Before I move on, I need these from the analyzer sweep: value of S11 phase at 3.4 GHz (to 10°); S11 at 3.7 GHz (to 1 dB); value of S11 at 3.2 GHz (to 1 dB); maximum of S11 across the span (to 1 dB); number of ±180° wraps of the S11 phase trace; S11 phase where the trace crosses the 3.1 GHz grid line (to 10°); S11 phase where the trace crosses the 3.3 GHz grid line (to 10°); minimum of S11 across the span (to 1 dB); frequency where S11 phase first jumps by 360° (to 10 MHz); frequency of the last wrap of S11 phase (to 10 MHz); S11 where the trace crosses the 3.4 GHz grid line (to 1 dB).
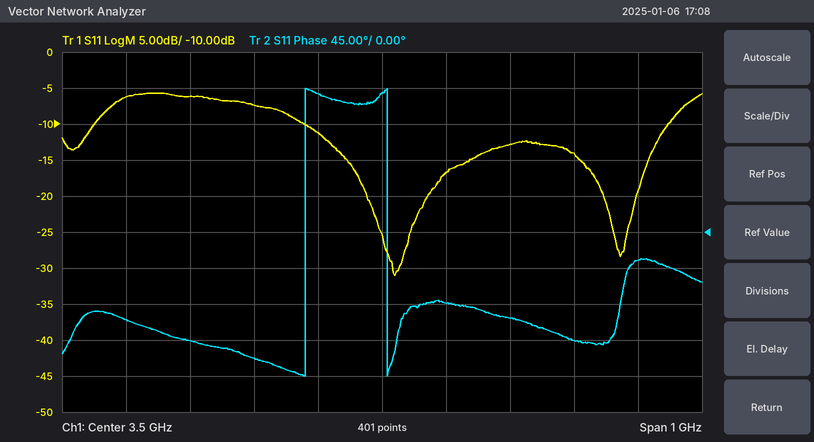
170°
-13 dB
-6 dB
-6 dB
2
-110°
-160°
-31 dB
3.38 GHz
3.51 GHz
-11 dB
